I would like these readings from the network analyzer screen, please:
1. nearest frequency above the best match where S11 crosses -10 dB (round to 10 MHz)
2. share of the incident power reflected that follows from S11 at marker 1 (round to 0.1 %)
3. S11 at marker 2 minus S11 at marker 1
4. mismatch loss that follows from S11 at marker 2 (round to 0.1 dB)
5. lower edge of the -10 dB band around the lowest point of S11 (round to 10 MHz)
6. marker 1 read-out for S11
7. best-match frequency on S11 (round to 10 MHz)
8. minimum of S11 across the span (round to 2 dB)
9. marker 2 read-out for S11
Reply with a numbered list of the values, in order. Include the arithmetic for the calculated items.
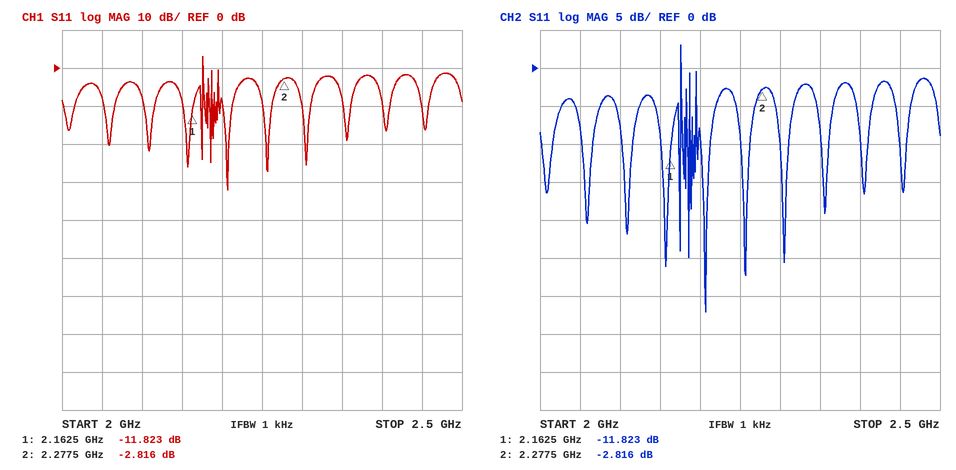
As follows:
1. 2.21 GHz
2. 10^(-11.823/10) ≈ 6.6 %
3. -2.816 − (-11.823) = 9.007 dB
4. −10 log10(1 − 10^(-2.816/10)) ≈ 3.2 dB
5. 2.20 GHz
6. -11.823 dB
7. 2.21 GHz
8. -32 dB
9. -2.816 dB
